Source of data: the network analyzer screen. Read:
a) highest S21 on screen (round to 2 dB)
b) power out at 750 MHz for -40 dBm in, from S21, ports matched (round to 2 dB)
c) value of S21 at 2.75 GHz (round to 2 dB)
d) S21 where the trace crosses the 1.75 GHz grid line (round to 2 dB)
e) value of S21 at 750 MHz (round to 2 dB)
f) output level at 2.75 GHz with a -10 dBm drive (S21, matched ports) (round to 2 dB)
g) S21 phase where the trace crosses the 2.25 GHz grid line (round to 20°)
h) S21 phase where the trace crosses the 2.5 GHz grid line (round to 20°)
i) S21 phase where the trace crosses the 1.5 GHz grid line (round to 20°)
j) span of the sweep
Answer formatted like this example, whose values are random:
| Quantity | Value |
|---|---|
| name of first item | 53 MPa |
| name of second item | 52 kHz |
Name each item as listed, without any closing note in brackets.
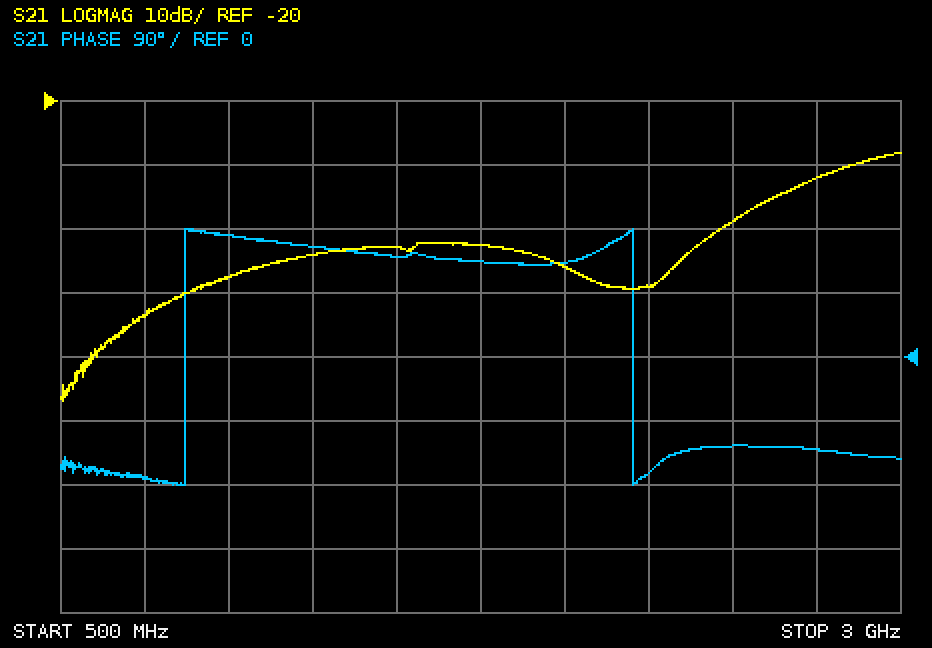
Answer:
| Quantity | Value |
|---|---|
| highest S21 on screen | -28 dB |
| power out at 750 MHz for -40 dBm in, from S21, ports matched | -94 dBm |
| value of S21 at 2.75 GHz | -32 dB |
| S21 where the trace crosses the 1.75 GHz grid line | -42 dB |
| value of S21 at 750 MHz | -54 dB |
| output level at 2.75 GHz with a -10 dBm drive (S21, matched ports) | -42 dBm |
| S21 phase where the trace crosses the 2.25 GHz grid line | -160° |
| S21 phase where the trace crosses the 2.5 GHz grid line | -120° |
| S21 phase where the trace crosses the 1.5 GHz grid line | 140° |
| span of the sweep | 2.5 GHz |
